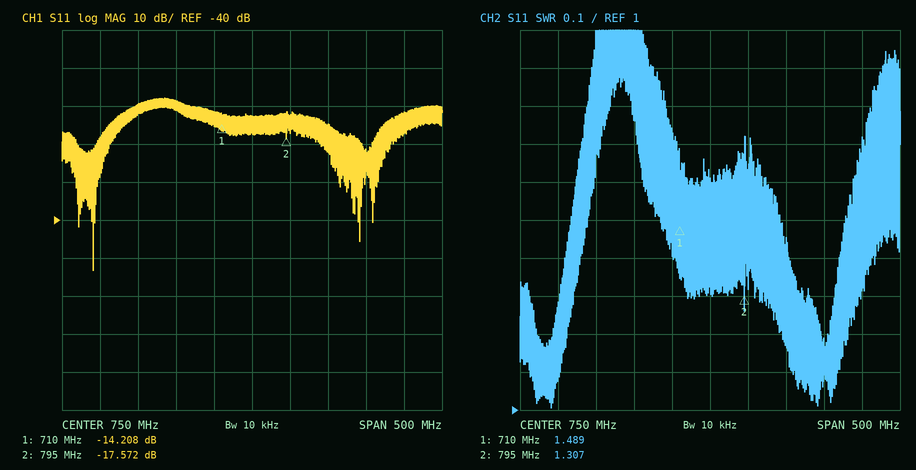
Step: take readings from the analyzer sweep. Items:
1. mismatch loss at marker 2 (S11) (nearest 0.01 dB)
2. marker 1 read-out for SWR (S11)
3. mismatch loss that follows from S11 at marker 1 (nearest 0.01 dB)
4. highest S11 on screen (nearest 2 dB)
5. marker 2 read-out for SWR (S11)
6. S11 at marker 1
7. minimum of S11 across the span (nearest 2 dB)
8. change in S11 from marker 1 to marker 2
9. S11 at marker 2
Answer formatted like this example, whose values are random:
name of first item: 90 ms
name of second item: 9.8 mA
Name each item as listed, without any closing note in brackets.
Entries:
mismatch loss at marker 2 (S11): 0.08 dB
marker 1 read-out for SWR: 1.489
mismatch loss that follows from S11 at marker 1: 0.17 dB
highest S11 on screen: -8 dB
marker 2 read-out for SWR: 1.307
S11 at marker 1: -14.208 dB
minimum of S11 across the span: -54 dB
change in S11 from marker 1 to marker 2: -3.364 dB
S11 at marker 2: -17.572 dB
